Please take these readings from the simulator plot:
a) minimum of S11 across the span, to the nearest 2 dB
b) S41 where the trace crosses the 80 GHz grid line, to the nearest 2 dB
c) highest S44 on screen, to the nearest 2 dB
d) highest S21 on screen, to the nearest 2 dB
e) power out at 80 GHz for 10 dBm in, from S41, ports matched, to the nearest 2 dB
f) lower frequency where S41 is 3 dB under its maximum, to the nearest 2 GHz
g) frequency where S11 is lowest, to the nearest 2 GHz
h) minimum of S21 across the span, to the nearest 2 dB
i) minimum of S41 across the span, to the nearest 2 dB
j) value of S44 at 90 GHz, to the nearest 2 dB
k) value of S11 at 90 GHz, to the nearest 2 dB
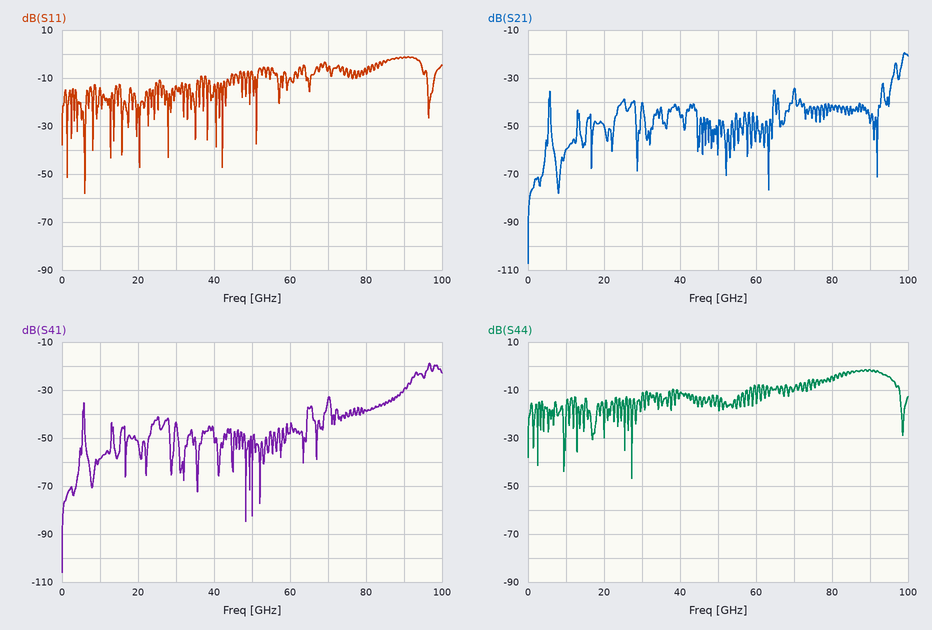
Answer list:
-58 dB
-38 dB
-2 dB
-20 dB
-28 dBm
96 GHz
6 GHz
-108 dB
-106 dB
-2 dB
-2 dB
